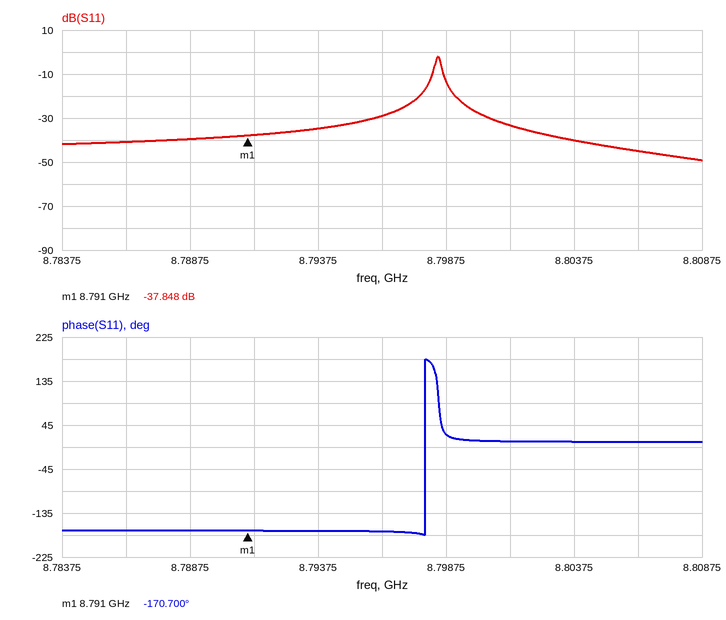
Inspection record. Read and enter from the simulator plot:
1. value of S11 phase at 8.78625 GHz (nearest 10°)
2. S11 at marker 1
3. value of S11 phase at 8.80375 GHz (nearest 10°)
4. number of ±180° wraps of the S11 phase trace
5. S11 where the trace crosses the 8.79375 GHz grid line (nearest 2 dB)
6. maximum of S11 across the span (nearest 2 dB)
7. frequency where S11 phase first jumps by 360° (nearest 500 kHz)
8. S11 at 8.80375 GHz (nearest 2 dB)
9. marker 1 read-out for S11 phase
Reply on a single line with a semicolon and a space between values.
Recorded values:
-170°; -37.848 dB; 10°; 1; -34 dB; -2 dB; 8.7980 GHz; -40 dB; -170.700°
